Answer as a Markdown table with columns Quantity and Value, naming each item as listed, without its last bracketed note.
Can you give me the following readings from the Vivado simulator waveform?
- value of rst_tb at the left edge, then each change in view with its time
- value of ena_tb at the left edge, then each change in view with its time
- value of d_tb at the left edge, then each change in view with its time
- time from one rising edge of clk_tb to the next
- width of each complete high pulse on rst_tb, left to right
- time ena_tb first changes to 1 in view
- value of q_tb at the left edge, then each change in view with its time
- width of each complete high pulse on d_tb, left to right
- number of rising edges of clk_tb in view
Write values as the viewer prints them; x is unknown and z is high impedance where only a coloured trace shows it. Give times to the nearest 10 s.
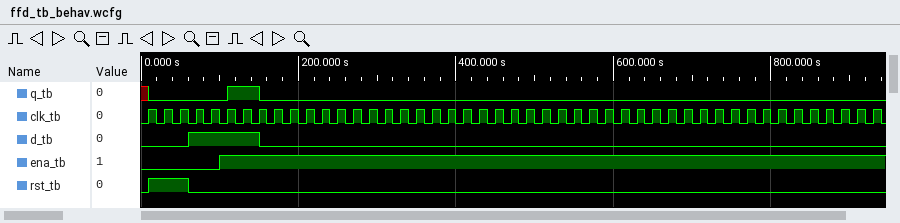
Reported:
| Quantity | Value |
|---|---|
| value of rst_tb at the left edge, then each change in view with its time | 0, 1 at 10 s, 0 at 60 s |
| value of ena_tb at the left edge, then each change in view with its time | 0, 1 at 100 s |
| value of d_tb at the left edge, then each change in view with its time | 0, 1 at 60 s, 0 at 150 s |
| time from one rising edge of clk_tb to the next | 20 s |
| width of each complete high pulse on rst_tb, left to right | 50 s |
| time ena_tb first changes to 1 in view | 100 s |
| value of q_tb at the left edge, then each change in view with its time | x, 0 at 10 s, 1 at 110 s, 0 at 150 s |
| width of each complete high pulse on d_tb, left to right | 90 s |
| number of rising edges of clk_tb in view | 47 |
